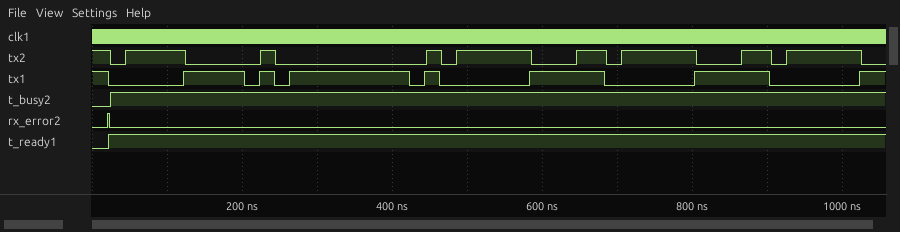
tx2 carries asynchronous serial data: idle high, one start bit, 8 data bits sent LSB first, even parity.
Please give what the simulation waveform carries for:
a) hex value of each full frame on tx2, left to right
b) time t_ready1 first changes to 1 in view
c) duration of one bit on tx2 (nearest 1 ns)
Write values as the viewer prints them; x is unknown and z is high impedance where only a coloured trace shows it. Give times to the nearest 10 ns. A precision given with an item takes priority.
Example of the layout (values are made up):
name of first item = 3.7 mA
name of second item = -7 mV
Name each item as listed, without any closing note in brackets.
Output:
hex value of each full frame on tx2, left to right = 0F, 00, 1F, 1F
time t_ready1 first changes to 1 in view = 20 ns
duration of one bit on tx2 = 20 ns
